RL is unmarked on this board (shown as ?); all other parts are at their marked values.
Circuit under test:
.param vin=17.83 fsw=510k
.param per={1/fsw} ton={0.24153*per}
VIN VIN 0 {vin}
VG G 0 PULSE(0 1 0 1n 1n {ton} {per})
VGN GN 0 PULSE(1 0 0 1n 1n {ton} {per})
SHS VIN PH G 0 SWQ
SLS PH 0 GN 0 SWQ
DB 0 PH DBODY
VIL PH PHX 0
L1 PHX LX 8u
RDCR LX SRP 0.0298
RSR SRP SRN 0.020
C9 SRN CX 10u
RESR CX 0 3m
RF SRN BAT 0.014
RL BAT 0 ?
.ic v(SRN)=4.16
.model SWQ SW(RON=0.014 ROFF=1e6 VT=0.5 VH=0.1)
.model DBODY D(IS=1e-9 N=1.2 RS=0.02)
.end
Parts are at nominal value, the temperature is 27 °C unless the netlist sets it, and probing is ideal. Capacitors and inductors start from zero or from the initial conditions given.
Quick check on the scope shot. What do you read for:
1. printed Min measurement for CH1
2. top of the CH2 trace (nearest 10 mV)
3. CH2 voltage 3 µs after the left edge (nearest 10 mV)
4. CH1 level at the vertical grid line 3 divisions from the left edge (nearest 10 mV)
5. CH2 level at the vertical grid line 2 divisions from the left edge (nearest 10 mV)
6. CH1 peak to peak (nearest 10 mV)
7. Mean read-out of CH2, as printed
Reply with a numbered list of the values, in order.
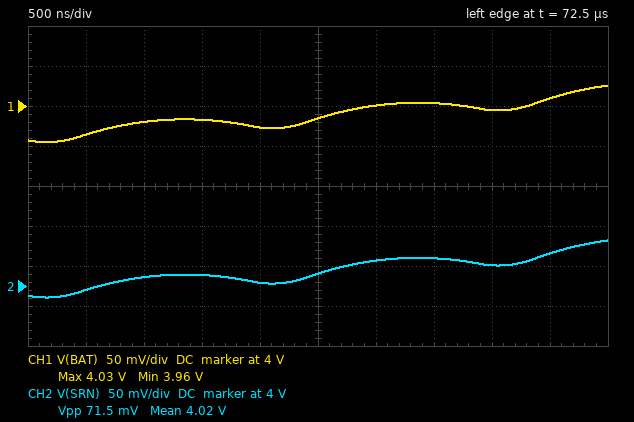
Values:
1. 3.96 V
2. 4.06 V
3. 4.03 V
4. 3.98 V
5. 4.01 V
6. 70 mV
7. 4.02 V
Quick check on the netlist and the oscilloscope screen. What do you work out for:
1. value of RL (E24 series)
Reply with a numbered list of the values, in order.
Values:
1. 1.8 Ω
